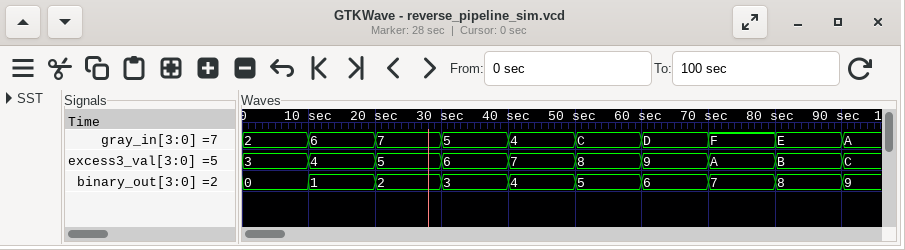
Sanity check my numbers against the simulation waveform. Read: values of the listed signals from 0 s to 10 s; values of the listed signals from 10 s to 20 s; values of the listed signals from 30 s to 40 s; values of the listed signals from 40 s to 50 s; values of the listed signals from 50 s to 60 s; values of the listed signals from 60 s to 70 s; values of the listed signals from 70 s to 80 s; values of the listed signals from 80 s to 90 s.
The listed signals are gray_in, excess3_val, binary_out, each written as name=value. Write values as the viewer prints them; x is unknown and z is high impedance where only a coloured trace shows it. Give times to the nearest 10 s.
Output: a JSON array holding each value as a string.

["gray_in=2, excess3_val=3, binary_out=0", "gray_in=6, excess3_val=4, binary_out=1", "gray_in=5, excess3_val=6, binary_out=3", "gray_in=4, excess3_val=7, binary_out=4", "gray_in=C, excess3_val=8, binary_out=5", "gray_in=D, excess3_val=9, binary_out=6", "gray_in=F, excess3_val=A, binary_out=7", "gray_in=E, excess3_val=B, binary_out=8"]
